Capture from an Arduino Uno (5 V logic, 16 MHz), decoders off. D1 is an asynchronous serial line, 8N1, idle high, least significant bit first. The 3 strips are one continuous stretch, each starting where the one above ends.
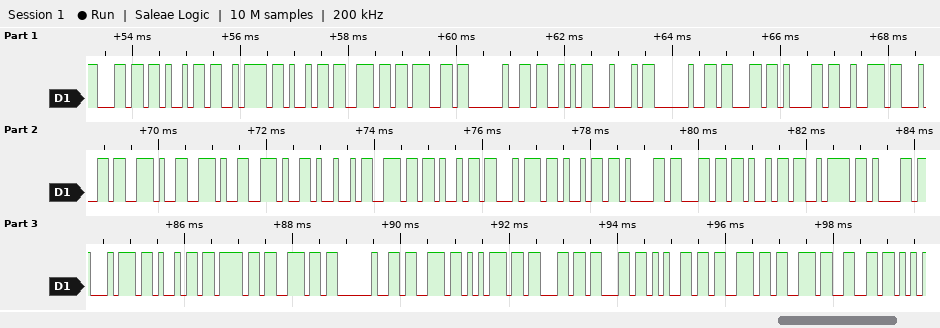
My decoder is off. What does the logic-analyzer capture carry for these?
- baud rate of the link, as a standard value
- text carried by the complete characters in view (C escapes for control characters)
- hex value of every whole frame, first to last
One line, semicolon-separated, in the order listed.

9600 baud; "lizing SD card...Initialization successf"; 6C 69 7A 69 6E 67 20 53 44 20 63 61 72 64 2E 2E 2E 49 6E 69 74 69 61 6C 69 7A 61 74 69 6F 6E 20 73 75 63 63 65 73 73 66
